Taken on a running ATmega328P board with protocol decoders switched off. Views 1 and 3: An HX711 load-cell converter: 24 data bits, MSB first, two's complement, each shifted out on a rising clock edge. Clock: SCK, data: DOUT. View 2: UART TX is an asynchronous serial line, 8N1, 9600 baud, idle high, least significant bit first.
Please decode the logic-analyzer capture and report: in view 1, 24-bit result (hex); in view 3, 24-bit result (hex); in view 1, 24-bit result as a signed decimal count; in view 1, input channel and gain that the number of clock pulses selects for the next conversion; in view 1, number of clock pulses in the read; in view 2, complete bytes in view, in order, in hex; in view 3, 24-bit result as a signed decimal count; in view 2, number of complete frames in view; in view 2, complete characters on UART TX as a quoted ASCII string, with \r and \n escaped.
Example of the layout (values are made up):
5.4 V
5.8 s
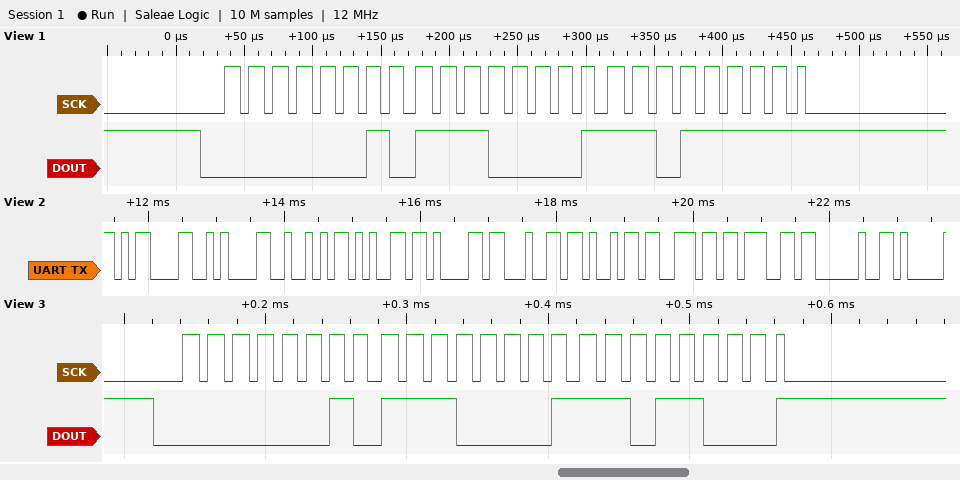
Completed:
0x02E1DF
0x02E1D8
188895
channel A, gain 128
25
0x0D 0x0A 0x52 0x65 0x61 0x64 0x69 0x6E 0x67 0x20
188888
10
"\r\nReading "
